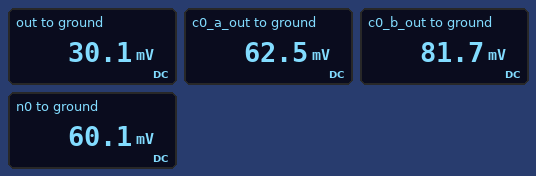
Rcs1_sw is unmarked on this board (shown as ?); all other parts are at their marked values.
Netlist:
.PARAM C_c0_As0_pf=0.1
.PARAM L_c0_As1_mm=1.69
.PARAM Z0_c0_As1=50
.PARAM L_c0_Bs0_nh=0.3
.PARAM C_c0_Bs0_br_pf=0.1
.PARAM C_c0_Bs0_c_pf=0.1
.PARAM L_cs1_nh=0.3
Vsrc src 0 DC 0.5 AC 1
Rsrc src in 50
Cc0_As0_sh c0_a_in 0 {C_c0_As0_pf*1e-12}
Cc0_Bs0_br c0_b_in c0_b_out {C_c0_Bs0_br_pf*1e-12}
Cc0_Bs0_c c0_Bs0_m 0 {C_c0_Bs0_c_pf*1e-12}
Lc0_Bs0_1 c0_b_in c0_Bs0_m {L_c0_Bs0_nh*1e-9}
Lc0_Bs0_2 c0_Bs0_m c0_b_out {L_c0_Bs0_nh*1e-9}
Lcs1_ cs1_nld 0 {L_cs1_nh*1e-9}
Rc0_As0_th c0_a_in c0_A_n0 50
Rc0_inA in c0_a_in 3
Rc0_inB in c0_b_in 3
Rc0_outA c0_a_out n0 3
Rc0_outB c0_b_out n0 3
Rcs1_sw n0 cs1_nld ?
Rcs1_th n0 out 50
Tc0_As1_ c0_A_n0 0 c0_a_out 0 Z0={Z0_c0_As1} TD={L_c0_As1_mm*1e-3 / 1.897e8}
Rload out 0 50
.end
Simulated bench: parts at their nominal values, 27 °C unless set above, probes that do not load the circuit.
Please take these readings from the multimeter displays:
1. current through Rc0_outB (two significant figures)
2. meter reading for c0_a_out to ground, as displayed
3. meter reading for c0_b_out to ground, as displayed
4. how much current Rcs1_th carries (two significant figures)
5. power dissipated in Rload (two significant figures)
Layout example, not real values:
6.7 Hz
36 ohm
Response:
7.2 mA
62.5 mV
81.7 mV
600 µA
18 µW
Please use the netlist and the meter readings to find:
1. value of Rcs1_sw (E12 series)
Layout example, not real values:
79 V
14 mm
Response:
8.2 Ω
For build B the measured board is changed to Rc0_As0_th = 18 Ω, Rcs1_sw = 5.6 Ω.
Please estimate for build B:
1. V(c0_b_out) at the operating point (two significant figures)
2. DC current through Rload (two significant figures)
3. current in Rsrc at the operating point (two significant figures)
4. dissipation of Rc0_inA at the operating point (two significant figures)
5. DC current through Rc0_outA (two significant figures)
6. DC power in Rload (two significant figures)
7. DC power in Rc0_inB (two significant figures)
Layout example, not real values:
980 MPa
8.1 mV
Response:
64 mV
440 µA
8.3 mA
8.3 µW
1.7 mA
9.7 µW
130 µW
